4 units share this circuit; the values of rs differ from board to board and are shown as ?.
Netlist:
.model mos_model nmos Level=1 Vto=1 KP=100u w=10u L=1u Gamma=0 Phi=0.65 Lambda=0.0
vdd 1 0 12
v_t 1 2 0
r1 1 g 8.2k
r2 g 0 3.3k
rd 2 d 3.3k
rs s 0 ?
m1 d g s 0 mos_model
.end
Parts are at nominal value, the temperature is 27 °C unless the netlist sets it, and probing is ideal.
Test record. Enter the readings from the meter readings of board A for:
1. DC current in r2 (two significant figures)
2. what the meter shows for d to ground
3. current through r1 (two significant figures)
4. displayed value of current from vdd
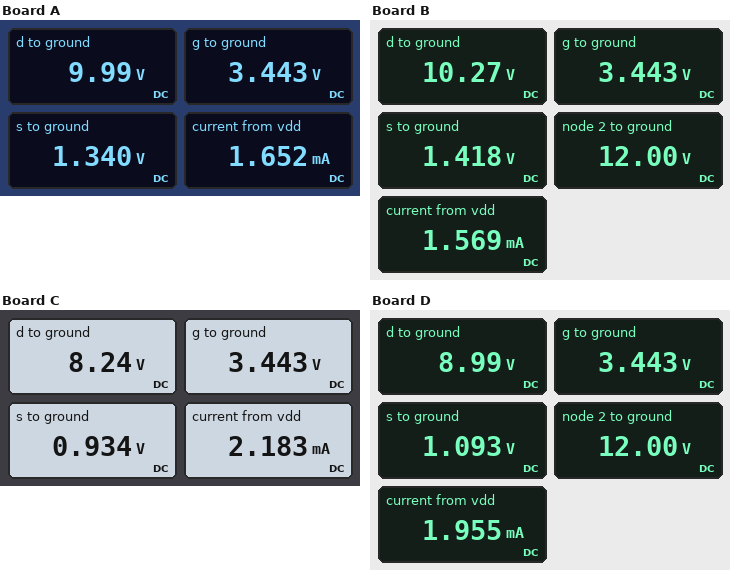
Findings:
1.0 mA
9.99 V
1.0 mA
1.652 mA
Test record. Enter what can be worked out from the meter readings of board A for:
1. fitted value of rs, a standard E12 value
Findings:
2.2 kΩ
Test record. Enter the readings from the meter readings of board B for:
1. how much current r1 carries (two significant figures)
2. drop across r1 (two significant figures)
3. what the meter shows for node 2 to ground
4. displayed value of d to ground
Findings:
1.0 mA
8.6 V
12.00 V
10.27 V
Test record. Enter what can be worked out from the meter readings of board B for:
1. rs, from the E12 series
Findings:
2.7 kΩ
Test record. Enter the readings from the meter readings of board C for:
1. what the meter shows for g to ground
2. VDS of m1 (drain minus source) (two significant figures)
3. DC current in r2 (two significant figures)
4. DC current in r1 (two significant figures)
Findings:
3.443 V
7.3 V
1.0 mA
1.0 mA
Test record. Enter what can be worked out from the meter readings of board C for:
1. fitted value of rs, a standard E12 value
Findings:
820 Ω
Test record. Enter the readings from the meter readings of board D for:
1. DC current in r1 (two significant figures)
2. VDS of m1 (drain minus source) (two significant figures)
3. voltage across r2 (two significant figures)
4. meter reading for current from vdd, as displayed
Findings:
1.0 mA
7.9 V
3.4 V
1.955 mA
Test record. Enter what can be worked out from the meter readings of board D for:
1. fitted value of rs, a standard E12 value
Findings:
1.2 kΩ
